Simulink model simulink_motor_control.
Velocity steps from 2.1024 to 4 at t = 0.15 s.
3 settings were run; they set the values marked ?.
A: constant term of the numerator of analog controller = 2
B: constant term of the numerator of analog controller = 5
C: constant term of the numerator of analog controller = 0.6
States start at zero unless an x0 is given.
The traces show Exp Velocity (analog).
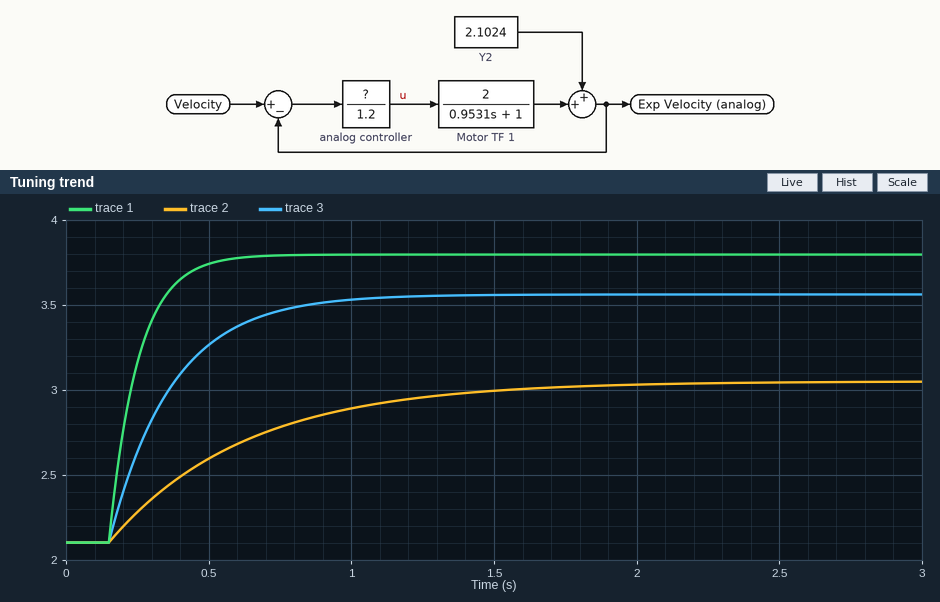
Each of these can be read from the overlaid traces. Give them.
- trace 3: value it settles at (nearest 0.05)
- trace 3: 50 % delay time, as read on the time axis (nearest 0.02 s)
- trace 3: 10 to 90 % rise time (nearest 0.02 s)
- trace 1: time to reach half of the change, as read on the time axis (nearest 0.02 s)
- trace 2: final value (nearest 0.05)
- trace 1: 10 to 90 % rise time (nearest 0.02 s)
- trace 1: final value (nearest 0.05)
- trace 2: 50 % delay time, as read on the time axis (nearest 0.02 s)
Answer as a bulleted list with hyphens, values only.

- 3.55
- 0.30 s
- 0.48 s
- 0.22 s
- 3.05
- 0.22 s
- 3.80
- 0.48 s
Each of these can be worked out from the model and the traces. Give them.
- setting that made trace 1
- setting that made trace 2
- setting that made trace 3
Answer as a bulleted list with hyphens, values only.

- B
- C
- A
